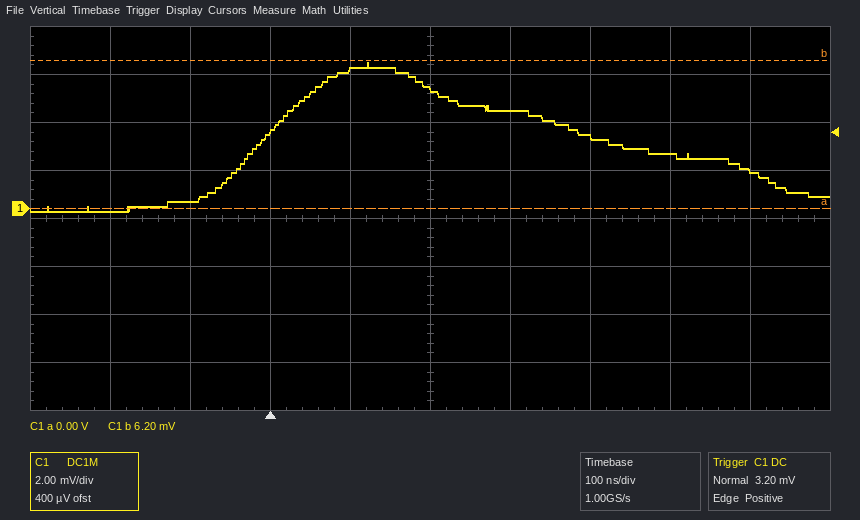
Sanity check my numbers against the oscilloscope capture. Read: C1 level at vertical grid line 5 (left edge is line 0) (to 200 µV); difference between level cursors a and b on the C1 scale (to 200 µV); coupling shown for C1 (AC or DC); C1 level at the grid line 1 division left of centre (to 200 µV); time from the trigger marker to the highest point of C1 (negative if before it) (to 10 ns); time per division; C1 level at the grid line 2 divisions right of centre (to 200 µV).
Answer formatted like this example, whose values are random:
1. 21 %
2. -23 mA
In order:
1. 5.0 mV
2. 6.2 mV
3. DC
4. 5.8 mV
5. +120 ns
6. 100 ns
7. 3.0 mV
